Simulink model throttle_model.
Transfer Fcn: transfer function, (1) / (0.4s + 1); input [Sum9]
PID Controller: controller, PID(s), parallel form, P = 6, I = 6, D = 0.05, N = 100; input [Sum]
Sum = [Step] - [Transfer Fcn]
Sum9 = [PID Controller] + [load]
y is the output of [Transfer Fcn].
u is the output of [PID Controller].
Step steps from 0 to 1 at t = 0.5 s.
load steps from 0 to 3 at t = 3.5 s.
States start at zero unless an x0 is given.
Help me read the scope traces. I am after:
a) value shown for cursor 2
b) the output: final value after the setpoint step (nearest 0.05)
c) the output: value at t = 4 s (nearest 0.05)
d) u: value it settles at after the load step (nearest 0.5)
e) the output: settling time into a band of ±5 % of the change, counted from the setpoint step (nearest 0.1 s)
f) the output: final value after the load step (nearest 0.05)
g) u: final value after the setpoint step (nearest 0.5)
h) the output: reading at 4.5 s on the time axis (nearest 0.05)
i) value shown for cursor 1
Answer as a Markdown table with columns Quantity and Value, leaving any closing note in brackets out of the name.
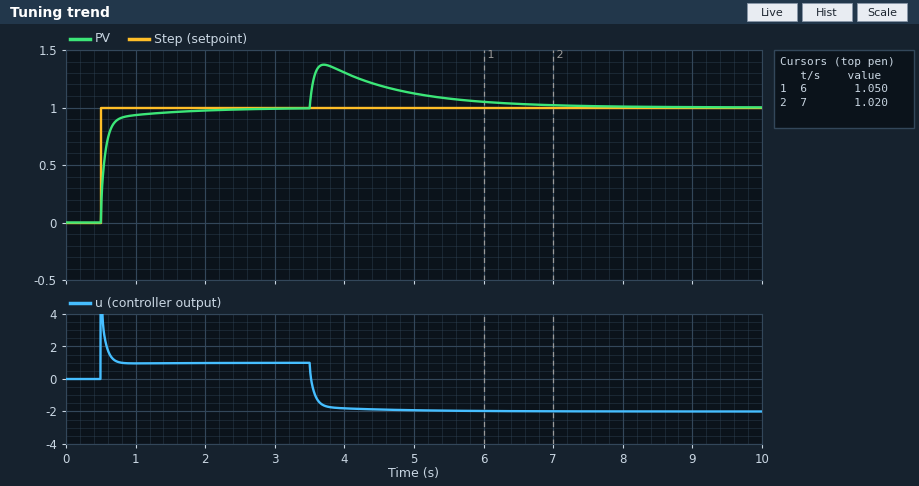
| Quantity | Value |
|---|---|
| value shown for cursor 2 | 1.020 |
| the output: final value after the setpoint step | 1.00 |
| the output: value at t = 4 s | 1.30 |
| u: value it settles at after the load step | -2.0 |
| the output: settling time into a band of ±5 % of the change, counted from the setpoint step | 0.8 s |
| the output: final value after the load step | 1.00 |
| u: final value after the setpoint step | 1.0 |
| the output: reading at 4.5 s on the time axis | 1.20 |
| value shown for cursor 1 | 1.050 |
